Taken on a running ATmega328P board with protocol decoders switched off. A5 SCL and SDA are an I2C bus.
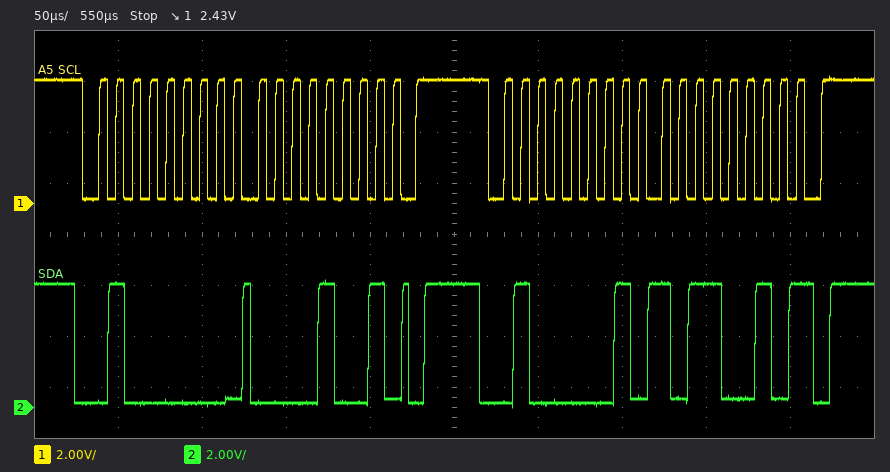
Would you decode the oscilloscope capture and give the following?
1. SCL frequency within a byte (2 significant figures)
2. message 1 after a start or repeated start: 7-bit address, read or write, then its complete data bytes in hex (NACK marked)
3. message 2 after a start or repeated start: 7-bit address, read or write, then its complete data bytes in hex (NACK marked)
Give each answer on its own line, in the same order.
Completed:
100 kHz
0x20 write: 09
0x20 read: B2 NACK
